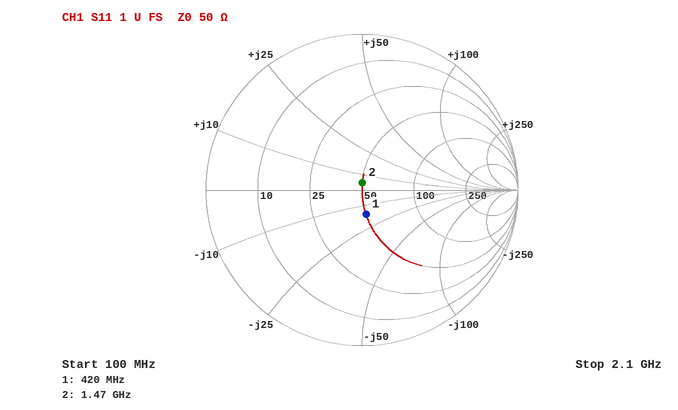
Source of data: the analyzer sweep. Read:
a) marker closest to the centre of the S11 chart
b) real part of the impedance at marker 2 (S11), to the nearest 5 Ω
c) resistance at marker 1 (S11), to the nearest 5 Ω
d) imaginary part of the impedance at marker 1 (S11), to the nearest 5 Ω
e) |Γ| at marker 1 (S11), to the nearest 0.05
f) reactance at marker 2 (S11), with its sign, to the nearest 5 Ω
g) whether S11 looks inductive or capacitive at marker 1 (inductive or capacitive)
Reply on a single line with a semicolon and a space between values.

marker 2; 50 Ω; 50 Ω; -15 Ω; 0.15; +5 Ω; capacitive
